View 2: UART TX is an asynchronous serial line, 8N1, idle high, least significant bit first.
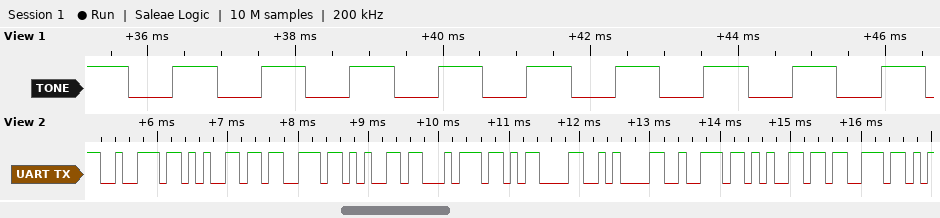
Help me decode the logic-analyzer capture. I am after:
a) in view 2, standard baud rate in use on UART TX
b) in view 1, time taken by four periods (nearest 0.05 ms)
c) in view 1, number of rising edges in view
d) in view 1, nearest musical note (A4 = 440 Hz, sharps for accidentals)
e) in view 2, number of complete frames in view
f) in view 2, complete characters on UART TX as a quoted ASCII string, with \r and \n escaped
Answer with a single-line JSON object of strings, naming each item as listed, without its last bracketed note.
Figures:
{"in view 2, standard baud rate in use on UART TX": "9600 baud", "in view 1, time taken by four periods": "4.80 ms", "in view 1, number of rising edges in view": "9", "in view 1, nearest musical note": "G#5", "in view 2, number of complete frames in view": "10", "in view 2, complete characters on UART TX as a quoted ASCII string, with \\r and \\n escaped": "\"reset\\r\\nres\""}
